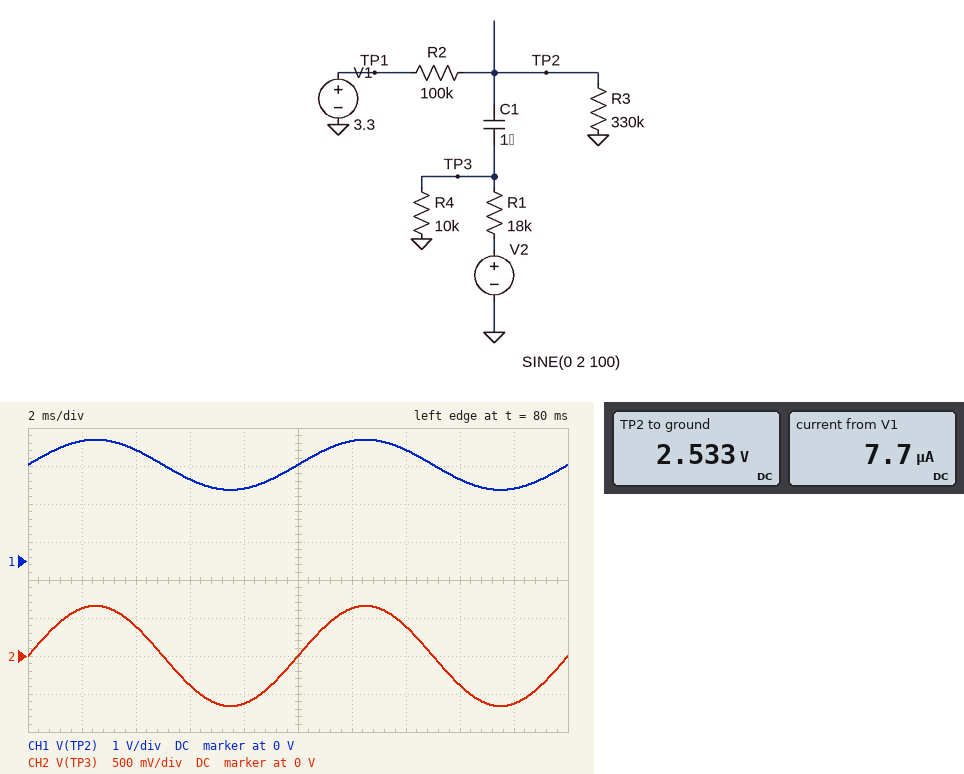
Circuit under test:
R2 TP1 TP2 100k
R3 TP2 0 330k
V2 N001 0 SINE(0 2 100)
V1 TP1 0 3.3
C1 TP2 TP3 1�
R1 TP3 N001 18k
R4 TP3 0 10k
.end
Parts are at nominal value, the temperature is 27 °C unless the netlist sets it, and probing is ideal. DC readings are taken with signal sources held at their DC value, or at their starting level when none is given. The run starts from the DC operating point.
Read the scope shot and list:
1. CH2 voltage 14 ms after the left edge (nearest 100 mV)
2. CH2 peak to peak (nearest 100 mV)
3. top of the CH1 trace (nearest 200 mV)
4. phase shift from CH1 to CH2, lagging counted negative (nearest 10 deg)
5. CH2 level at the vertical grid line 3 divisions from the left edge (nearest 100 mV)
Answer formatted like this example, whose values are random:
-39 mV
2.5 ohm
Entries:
400 mV
1.3 V
3.2 V
0 deg
-400 mV
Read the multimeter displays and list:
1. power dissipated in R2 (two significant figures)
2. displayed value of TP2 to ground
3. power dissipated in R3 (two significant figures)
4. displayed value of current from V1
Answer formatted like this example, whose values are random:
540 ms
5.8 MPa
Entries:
5.9 µW
2.533 V
19 µW
7.7 µA
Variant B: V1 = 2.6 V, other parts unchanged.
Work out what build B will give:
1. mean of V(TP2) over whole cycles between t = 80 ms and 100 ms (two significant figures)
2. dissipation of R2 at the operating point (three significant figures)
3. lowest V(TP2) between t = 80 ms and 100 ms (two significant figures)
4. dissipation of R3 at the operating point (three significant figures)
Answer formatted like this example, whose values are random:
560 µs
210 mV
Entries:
2.0 V
3.66 µW
1.3 V
12.1 µW
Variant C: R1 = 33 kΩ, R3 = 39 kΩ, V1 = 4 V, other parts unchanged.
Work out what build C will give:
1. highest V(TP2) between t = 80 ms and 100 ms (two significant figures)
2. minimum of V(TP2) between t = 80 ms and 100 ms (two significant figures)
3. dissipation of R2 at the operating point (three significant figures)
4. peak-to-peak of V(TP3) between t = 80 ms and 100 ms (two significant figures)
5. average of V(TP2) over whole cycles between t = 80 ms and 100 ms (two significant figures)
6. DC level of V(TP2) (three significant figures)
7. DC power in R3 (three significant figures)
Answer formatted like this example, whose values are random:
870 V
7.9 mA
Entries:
1.5 V
760 mV
82.8 µW
730 mV
1.1 V
1.12 V
32.3 µW
